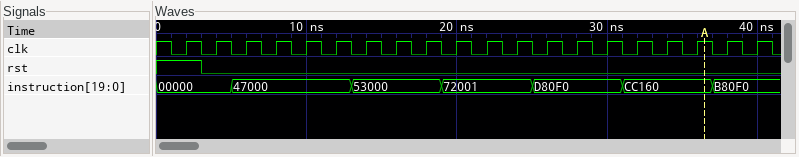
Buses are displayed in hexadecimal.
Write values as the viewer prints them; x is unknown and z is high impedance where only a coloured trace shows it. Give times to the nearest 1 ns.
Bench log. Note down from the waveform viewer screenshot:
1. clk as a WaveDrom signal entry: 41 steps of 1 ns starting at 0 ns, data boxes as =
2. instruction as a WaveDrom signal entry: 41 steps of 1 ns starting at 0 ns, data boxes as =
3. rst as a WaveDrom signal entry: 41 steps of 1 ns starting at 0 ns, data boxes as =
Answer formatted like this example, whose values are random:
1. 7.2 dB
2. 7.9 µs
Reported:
1. {name: 'clk', wave: '10101010101010101010101010101010101010101'}
2. {name: 'instruction', wave: '=....=.......=.....=.....=.....=.....=...', data: '00000 47000 53000 72001 D80F0 CC160 B80F0'}
3. {name: 'rst', wave: '1..0.....................................'}
